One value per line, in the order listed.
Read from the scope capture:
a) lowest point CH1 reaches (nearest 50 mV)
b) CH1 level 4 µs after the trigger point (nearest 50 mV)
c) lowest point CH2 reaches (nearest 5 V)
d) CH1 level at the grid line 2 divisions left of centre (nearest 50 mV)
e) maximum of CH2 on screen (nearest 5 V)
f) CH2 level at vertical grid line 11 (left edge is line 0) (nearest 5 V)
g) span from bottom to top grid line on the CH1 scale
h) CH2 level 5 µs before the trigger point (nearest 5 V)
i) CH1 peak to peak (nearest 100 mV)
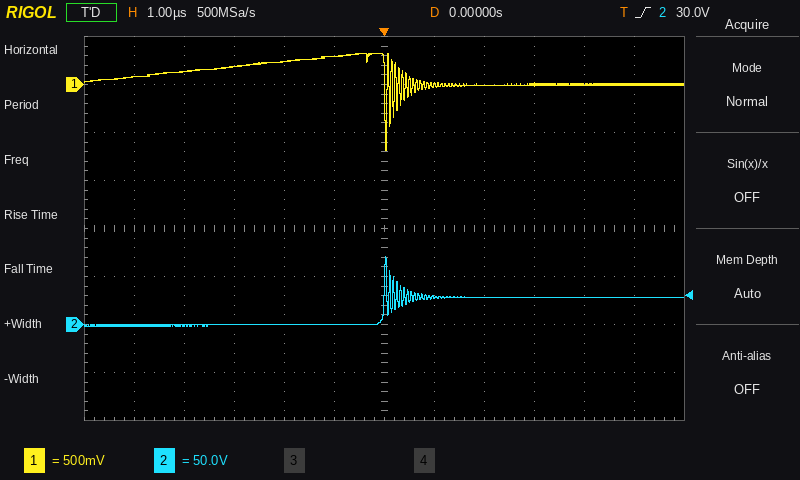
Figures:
-700 mV
0 mV
0 V
250 mV
70 V
30 V
4 V
0 V
1.00 V
